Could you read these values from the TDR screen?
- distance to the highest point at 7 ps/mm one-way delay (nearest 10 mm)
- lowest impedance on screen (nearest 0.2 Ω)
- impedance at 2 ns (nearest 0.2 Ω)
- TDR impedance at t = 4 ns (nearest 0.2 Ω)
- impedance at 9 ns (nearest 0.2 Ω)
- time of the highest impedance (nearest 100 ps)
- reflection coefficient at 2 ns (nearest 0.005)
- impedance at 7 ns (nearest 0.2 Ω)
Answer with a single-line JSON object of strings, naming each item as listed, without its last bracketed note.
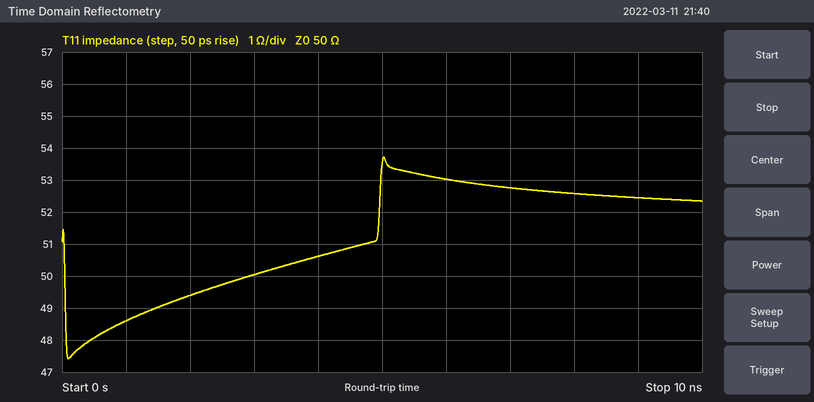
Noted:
{"distance to the highest point at 7 ps/mm one-way delay": "360 mm", "lowest impedance on screen": "47.4 Ω", "impedance at 2 ns": "49.4 Ω", "TDR impedance at t = 4 ns": "50.6 Ω", "impedance at 9 ns": "52.4 Ω", "time of the highest impedance": "5.0 ns", "reflection coefficient at 2 ns": "-0.005", "impedance at 7 ns": "52.8 Ω"}
